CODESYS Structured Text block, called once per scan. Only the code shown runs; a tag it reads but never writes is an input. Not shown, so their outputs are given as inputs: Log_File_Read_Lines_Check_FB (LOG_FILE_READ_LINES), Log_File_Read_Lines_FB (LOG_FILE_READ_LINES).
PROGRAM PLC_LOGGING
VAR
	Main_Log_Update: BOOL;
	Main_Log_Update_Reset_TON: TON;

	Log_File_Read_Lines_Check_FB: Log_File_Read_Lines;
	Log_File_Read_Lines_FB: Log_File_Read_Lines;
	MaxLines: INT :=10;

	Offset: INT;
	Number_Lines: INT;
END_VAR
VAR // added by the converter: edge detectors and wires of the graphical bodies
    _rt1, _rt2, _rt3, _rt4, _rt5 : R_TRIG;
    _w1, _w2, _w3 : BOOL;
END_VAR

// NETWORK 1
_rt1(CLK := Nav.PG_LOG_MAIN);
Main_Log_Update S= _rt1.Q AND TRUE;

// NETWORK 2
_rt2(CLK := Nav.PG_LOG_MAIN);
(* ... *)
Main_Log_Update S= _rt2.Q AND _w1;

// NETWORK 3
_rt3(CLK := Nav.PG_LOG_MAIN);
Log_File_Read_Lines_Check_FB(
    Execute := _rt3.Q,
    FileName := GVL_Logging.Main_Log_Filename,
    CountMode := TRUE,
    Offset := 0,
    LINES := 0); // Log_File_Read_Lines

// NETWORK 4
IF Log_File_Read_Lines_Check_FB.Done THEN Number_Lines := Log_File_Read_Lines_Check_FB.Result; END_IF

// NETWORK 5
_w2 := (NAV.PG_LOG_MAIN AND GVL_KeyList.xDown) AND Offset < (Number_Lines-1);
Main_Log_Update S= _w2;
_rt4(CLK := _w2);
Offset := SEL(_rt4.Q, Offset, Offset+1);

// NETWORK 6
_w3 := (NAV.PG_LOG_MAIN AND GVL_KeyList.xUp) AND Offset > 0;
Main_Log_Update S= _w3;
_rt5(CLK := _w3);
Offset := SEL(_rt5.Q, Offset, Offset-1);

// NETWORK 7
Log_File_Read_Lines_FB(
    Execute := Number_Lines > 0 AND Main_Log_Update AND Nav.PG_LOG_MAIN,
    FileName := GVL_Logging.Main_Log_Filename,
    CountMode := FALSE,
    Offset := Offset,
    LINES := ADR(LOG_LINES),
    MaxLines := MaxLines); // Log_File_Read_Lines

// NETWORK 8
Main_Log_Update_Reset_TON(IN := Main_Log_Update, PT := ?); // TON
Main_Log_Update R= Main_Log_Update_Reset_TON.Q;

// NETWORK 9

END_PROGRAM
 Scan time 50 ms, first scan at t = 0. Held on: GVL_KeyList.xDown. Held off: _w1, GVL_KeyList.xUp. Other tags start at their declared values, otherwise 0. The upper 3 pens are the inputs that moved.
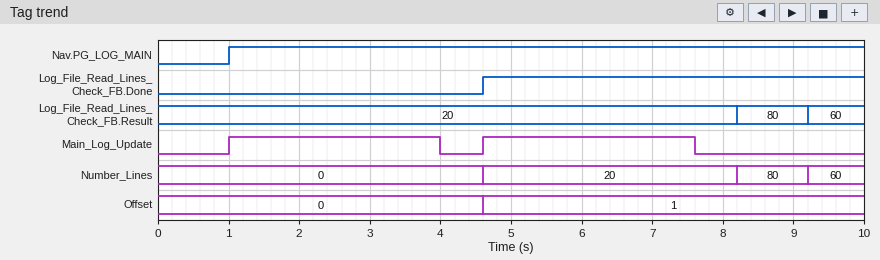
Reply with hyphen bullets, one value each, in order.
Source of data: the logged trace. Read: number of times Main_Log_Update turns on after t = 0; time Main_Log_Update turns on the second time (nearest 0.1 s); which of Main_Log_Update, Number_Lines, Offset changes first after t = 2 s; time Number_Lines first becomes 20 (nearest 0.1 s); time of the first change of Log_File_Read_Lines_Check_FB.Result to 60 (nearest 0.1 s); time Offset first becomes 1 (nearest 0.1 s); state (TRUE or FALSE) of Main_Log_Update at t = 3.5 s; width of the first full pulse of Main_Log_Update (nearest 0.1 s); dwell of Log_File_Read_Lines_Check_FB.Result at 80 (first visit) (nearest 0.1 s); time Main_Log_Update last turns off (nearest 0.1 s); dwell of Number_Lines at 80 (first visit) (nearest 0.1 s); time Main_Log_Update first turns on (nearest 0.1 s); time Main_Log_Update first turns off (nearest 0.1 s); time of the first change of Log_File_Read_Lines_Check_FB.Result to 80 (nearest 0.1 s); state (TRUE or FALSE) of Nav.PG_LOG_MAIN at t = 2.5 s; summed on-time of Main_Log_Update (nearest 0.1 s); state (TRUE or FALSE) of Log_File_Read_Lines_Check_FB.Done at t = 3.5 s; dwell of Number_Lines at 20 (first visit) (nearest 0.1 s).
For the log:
- 2
- 4.6 s
- Main_Log_Update
- 4.6 s
- 9.2 s
- 4.6 s
- TRUE
- 3.0 s
- 1.0 s
- 7.6 s
- 1.0 s
- 1.0 s
- 4.0 s
- 8.2 s
- TRUE
- 6.0 s
- FALSE
- 3.6 s
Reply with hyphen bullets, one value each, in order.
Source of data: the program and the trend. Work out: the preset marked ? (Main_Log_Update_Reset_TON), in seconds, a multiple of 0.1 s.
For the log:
- 3.0 s
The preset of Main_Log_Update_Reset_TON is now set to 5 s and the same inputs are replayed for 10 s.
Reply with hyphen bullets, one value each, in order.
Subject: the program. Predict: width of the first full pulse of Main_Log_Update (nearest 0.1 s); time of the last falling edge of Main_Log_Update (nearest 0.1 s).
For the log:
- 5.0 s
- 6.0 s
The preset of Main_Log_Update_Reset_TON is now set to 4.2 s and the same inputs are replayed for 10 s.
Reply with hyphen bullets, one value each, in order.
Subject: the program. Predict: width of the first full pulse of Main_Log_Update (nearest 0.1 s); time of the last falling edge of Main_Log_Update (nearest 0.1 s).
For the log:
- 4.2 s
- 5.2 s
